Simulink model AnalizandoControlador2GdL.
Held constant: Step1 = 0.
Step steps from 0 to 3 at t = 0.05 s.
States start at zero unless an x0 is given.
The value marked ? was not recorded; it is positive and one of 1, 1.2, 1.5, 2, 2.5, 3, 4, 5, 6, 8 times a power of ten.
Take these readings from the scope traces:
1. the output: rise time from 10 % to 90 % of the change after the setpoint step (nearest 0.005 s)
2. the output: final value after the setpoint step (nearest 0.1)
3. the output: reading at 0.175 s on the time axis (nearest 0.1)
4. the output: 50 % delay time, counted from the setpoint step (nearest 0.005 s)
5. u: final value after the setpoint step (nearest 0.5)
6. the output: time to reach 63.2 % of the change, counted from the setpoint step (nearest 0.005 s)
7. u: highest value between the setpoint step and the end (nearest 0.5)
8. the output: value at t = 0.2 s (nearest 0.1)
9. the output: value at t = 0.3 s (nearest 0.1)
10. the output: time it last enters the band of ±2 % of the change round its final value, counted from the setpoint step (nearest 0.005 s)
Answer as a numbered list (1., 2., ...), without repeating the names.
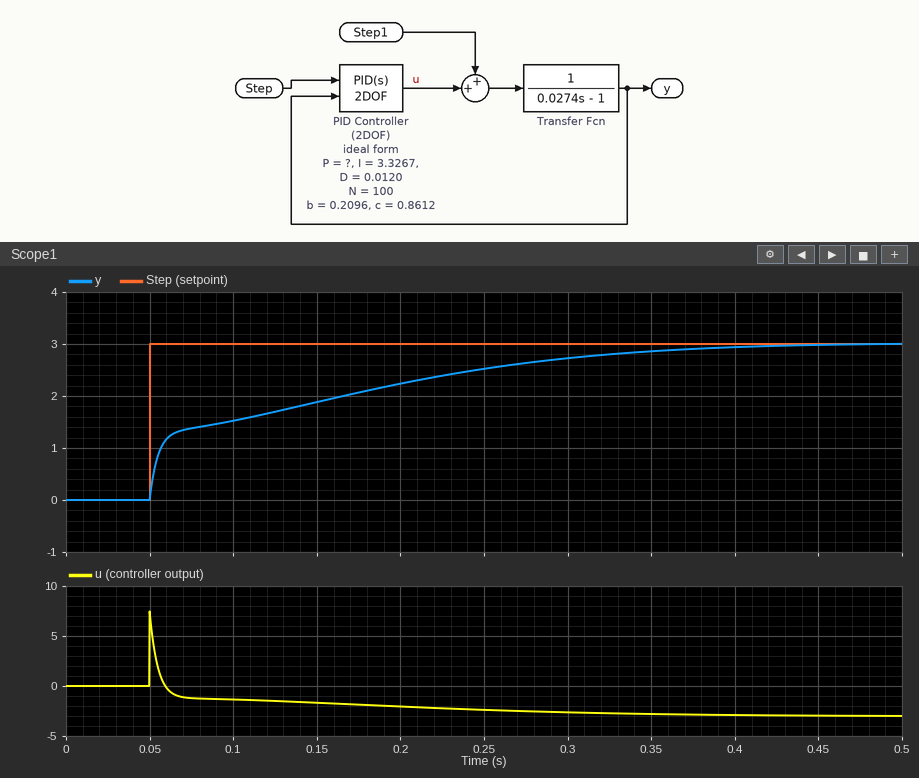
1. 0.240 s
2. 3.0
3. 2.1
4. 0.045 s
5. -3.0
6. 0.100 s
7. 7.5
8. 2.2
9. 2.7
10. 0.350 s
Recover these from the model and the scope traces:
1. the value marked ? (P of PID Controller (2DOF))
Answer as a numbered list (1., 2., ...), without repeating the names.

1. 2
